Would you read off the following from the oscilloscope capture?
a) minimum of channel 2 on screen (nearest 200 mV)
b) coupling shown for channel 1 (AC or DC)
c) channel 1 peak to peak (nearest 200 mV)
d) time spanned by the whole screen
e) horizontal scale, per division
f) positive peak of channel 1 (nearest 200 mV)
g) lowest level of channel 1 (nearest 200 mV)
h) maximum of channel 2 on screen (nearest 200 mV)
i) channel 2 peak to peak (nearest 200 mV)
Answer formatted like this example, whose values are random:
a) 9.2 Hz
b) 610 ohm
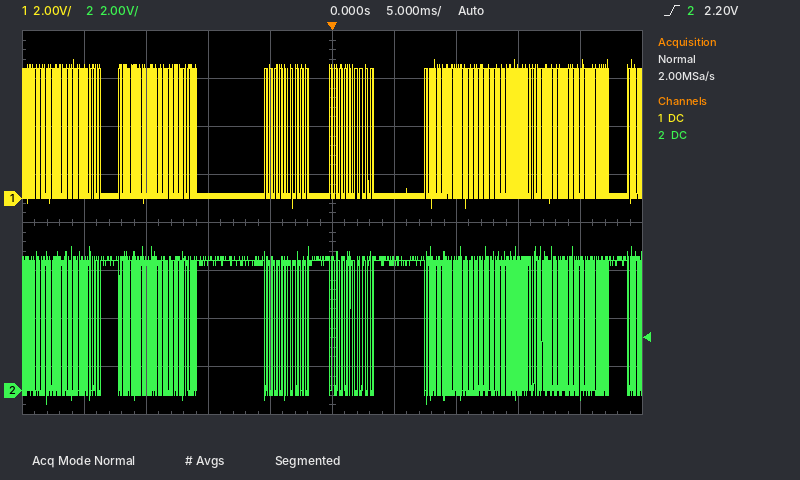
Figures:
a) -600 mV
b) DC
c) 6.2 V
d) 50 ms
e) 5 ms
f) 5.8 V
g) -400 mV
h) 6.0 V
i) 6.6 V
